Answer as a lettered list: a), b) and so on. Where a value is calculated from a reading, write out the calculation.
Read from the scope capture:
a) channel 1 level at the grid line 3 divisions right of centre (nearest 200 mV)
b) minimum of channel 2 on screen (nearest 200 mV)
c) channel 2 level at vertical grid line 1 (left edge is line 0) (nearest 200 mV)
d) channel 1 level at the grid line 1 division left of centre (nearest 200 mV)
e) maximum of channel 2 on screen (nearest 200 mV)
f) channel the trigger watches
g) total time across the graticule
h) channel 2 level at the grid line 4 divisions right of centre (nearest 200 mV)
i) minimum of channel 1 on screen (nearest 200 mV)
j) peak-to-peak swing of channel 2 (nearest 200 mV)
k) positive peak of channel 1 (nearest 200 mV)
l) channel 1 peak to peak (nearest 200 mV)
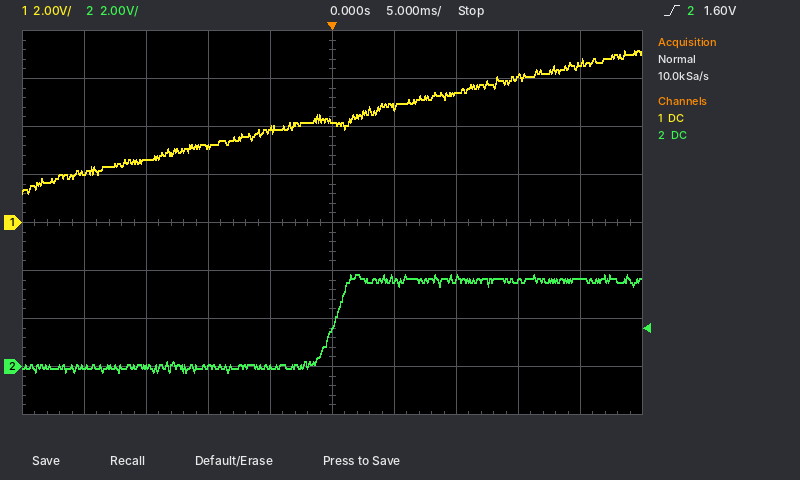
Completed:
a) 6.0 V
b) -200 mV
c) 0.0 V
d) 3.8 V
e) 3.8 V
f) channel 2
g) 50 ms
h) 3.6 V
i) 1.2 V
j) 3.8 V − (-200 mV) = 4.0 V
k) 7.2 V
l) 7.2 V − (1.2 V) = 6.0 V
